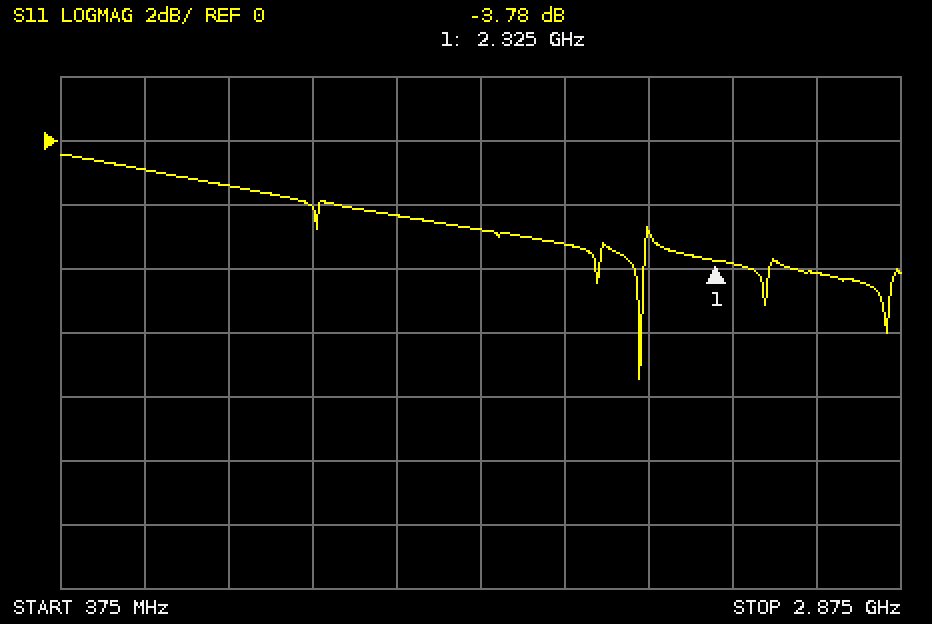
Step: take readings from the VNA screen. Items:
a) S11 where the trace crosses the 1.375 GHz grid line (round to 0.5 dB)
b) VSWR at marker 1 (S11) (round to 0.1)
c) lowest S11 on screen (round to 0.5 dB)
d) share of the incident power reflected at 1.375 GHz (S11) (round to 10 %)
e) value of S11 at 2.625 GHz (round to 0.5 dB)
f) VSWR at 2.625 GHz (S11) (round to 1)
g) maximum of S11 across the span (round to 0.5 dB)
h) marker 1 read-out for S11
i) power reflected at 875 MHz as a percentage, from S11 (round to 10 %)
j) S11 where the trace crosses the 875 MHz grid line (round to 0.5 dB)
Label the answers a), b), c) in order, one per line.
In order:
a) -2.5 dB
b) 4.7
c) -7.5 dB
d) 60 %
e) -4.0 dB
f) 4
g) -0.5 dB
h) -3.78 dB
i) 70 %
j) -1.5 dB
